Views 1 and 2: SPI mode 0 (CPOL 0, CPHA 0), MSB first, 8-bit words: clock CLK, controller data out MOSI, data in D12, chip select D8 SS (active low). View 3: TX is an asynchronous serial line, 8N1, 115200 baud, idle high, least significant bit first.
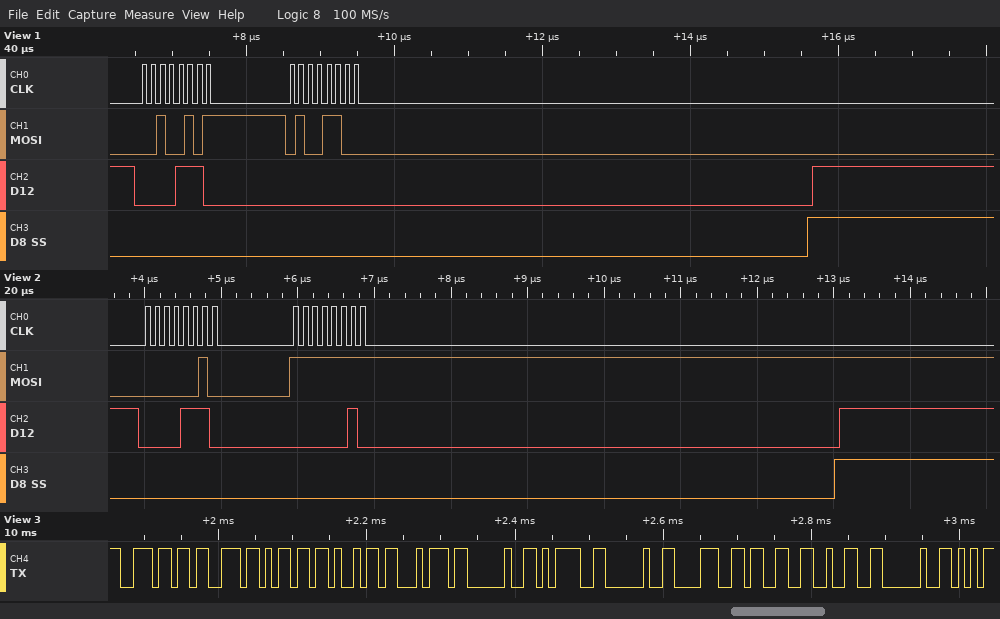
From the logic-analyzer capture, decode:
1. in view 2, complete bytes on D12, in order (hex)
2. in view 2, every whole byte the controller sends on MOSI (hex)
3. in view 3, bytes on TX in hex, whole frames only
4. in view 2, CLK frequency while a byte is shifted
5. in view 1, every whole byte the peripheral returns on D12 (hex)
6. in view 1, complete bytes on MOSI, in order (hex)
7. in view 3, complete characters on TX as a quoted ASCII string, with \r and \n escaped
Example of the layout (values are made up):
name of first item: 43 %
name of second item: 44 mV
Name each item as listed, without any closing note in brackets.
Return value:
in view 2, complete bytes on D12, in order: 0x0E 0x02
in view 2, every whole byte the controller sends on MOSI: 0x02 0xFF
in view 3, bytes on TX in hex, whole frames only: 6E 73 6D 69 74 20 3D 20 38 33 32 20
in view 2, CLK frequency while a byte is shifted: 8 MHz
in view 1, every whole byte the peripheral returns on D12: 0x0E 0x00
in view 1, complete bytes on MOSI, in order: 0x25 0x4C
in view 3, complete characters on TX as a quoted ASCII string, with \r and \n escaped: "nsmit = 832 "
